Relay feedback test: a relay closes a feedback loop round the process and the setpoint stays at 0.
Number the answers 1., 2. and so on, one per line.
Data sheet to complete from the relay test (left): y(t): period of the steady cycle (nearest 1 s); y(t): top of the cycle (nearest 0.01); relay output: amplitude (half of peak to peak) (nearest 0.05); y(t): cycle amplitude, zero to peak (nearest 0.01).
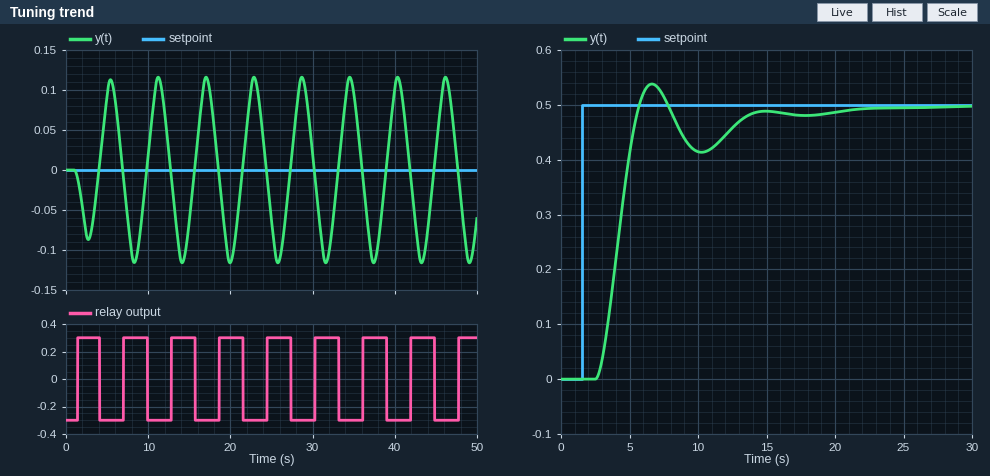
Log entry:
1. 6 s
2. 0.12
3. 0.30
4. 0.12
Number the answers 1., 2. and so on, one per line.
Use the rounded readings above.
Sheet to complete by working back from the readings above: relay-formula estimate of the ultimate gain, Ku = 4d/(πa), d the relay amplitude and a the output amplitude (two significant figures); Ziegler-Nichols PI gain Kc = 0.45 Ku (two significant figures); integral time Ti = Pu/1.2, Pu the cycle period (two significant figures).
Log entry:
1. 3.2
2. 1.4
3. 5.0 s
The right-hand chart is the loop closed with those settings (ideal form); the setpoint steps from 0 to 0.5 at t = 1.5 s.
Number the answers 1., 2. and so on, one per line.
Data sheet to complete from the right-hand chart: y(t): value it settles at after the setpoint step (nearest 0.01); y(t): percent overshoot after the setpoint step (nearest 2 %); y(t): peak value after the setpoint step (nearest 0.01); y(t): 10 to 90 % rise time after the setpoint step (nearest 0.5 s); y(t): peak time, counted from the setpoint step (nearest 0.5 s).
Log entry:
1. 0.50
2. 8 %
3. 0.54
4. 2.0 s
5. 5.0 s
